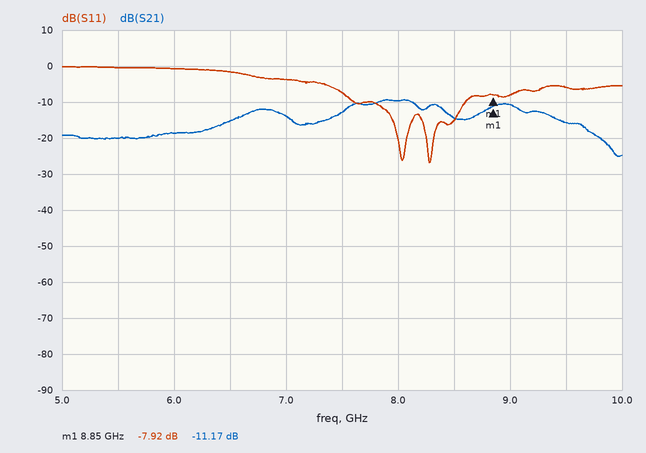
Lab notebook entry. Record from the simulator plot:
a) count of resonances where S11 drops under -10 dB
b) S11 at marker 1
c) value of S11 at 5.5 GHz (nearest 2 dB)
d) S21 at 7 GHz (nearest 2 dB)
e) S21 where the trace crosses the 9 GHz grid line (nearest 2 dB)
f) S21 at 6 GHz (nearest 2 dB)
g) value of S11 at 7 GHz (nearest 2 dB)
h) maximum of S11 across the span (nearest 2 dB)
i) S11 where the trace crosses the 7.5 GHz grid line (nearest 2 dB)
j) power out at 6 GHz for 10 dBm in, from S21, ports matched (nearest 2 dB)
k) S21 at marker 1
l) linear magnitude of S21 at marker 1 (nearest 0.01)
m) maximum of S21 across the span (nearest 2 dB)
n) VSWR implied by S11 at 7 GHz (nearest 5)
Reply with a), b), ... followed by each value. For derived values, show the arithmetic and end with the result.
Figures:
a) 2
b) -7.92 dB
c) 0 dB
d) -14 dB
e) -10 dB
f) -18 dB
g) -4 dB
h) 0 dB
i) -8 dB
j) 10 dBm + (-18 dB) = -8 dBm
k) -11.17 dB
l) 10^(-11.17/20) ≈ 0.28
m) -10 dB
n) |Γ| = 10^(-4/20) = 0.6310; VSWR = (1 + 0.6310)/(1 − 0.6310) ≈ 4.42, so 5 to the nearest 5
